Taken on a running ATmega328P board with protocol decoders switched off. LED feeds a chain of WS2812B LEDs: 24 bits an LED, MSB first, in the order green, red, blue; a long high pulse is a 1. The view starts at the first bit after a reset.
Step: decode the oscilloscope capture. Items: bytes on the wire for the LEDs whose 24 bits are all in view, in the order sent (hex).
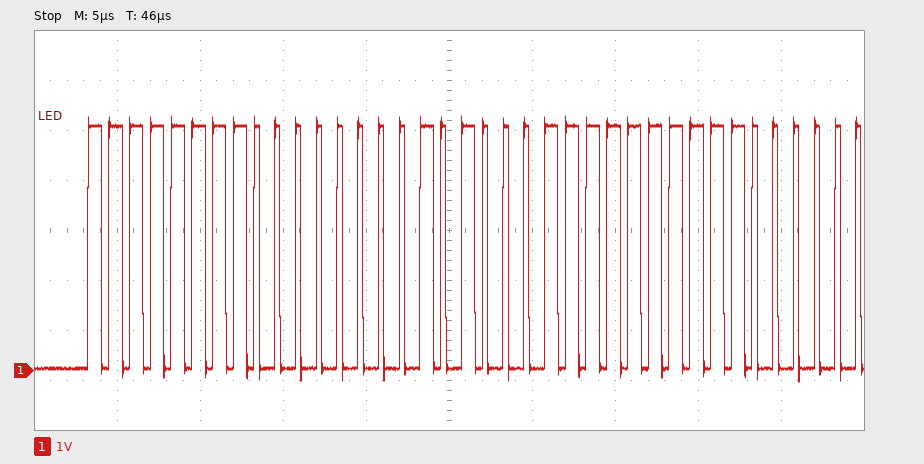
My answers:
FF 00 A3
